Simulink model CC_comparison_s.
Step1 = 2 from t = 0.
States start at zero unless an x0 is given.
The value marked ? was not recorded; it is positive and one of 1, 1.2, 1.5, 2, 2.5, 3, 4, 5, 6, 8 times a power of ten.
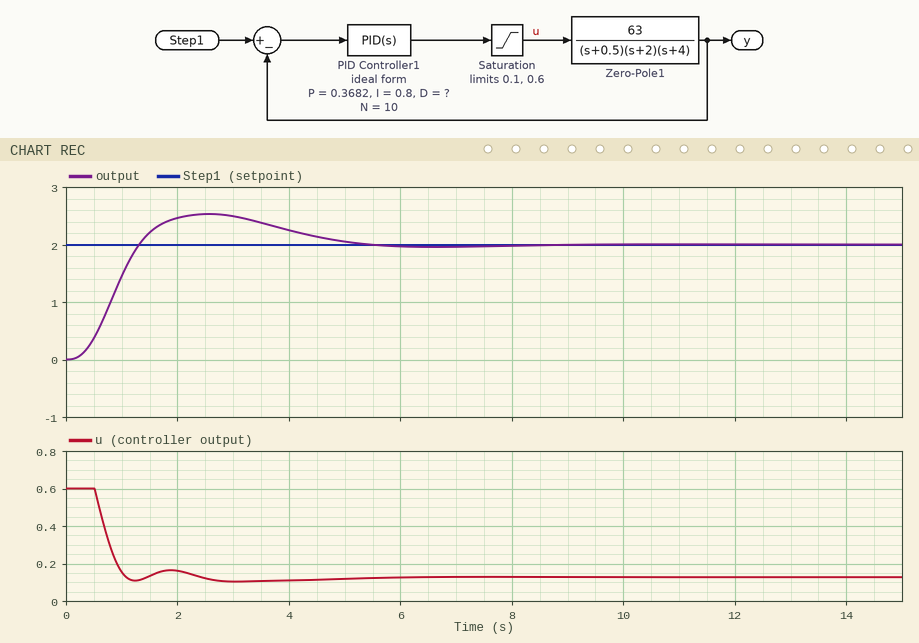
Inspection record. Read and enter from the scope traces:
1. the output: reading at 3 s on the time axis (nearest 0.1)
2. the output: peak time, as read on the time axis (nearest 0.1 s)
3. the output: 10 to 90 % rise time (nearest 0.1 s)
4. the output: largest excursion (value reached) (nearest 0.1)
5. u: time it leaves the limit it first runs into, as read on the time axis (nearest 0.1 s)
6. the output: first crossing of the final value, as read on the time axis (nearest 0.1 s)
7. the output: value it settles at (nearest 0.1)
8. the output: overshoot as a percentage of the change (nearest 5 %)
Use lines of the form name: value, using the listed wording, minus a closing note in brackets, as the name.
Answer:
the output: reading at 3 s on the time axis: 2.5
the output: peak time, as read on the time axis: 2.6 s
the output: 10 to 90 % rise time: 0.8 s
the output: largest excursion (value reached): 2.5
u: time it leaves the limit it first runs into, as read on the time axis: 0.5 s
the output: first crossing of the final value, as read on the time axis: 1.3 s
the output: value it settles at: 2.0
the output: overshoot as a percentage of the change: 25 %
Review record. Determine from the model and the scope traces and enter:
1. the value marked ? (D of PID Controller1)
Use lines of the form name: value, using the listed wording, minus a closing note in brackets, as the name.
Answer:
the value marked ?: 0.6
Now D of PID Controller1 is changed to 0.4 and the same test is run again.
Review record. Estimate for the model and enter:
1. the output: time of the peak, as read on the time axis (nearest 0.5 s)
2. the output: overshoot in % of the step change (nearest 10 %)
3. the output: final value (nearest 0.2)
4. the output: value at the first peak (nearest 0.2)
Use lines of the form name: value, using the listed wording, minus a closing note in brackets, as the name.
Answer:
the output: time of the peak, as read on the time axis: 2.0 s
the output: overshoot in % of the step change: 40 %
the output: final value: 2.0
the output: value at the first peak: 2.8
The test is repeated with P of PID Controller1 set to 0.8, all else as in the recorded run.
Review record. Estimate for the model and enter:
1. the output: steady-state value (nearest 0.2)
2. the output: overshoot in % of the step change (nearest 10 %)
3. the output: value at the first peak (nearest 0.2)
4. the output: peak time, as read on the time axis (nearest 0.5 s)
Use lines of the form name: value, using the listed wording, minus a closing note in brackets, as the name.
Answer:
the output: steady-state value: 2.0
the output: overshoot in % of the step change: 40 %
the output: value at the first peak: 2.8
the output: peak time, as read on the time axis: 2.0 s
